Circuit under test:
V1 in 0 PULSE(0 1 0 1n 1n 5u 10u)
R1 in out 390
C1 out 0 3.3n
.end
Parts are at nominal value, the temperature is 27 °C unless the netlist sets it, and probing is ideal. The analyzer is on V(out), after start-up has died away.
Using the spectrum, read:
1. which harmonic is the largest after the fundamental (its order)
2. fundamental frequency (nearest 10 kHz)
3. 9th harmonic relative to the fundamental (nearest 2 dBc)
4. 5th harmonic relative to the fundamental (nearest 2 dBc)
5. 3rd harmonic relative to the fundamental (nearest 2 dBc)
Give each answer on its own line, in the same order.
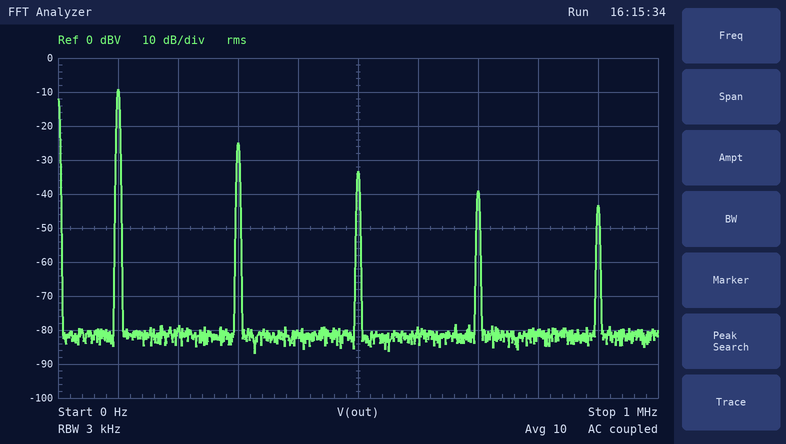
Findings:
3
100 kHz
-34 dBc
-24 dBc
-16 dBc
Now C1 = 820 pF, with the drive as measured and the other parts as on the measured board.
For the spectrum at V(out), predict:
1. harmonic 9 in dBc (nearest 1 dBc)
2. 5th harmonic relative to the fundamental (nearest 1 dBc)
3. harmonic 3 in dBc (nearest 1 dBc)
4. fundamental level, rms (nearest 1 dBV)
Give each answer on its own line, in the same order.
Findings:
-25 dBc
-17 dBc
-11 dBc
-7 dBV
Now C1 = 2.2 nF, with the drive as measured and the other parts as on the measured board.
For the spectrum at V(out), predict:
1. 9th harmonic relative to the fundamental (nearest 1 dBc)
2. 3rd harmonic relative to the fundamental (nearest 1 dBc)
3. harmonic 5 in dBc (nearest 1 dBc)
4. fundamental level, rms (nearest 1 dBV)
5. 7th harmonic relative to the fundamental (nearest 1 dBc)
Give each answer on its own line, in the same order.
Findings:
-32 dBc
-14 dBc
-22 dBc
-8 dBV
-28 dBc
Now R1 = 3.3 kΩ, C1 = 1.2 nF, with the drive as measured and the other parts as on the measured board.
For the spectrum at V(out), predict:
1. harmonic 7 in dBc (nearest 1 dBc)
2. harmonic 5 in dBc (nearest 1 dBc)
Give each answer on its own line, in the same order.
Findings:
-33 dBc
-27 dBc
